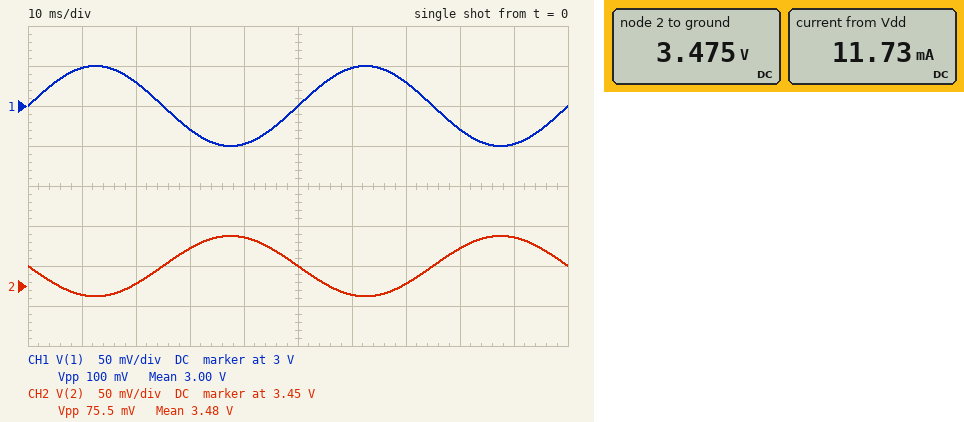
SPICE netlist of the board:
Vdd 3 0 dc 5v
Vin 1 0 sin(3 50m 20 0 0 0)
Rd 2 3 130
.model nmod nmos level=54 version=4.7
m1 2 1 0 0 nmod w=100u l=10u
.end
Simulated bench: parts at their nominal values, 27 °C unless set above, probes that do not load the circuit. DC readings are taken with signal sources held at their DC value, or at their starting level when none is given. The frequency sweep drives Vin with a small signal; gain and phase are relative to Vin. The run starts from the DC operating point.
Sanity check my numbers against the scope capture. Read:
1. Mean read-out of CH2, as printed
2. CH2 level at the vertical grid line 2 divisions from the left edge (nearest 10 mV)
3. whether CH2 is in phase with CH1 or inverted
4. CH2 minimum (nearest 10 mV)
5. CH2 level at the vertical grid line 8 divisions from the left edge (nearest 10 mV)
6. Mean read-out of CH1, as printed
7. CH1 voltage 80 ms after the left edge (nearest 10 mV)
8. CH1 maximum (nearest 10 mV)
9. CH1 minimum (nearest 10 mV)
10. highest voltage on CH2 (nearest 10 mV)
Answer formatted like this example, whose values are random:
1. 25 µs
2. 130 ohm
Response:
1. 3.48 V
2. 3.45 V
3. inverted
4. 3.44 V
5. 3.50 V
6. 3.00 V
7. 2.97 V
8. 3.05 V
9. 2.95 V
10. 3.51 V
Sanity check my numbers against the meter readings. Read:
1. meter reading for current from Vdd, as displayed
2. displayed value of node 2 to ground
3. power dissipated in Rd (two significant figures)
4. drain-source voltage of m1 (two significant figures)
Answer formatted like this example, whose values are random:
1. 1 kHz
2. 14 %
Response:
1. 11.73 mA
2. 3.475 V
3. 18 mW
4. 3.5 V
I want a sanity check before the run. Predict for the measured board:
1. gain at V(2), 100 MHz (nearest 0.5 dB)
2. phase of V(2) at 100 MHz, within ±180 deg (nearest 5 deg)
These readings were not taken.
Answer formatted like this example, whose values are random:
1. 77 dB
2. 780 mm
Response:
1. -2.0 dB
2. 160 deg
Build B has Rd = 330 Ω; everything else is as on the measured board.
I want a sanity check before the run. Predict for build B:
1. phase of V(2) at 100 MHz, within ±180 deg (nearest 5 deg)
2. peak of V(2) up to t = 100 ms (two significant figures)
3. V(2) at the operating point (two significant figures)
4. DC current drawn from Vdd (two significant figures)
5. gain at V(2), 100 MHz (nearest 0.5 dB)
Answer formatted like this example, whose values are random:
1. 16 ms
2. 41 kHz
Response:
1. 125 deg
2. 1.7 V
3. 1.6 V
4. 10 mA
5. -2.5 dB
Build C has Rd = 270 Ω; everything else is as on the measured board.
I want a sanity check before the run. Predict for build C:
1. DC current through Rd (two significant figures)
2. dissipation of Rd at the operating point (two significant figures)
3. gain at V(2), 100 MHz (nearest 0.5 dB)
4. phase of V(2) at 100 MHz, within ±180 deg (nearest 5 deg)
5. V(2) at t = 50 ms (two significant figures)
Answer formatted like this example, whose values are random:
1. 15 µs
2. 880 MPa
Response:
1. 11 mA
2. 33 mW
3. -0.5 dB
4. 140 deg
5. 2.0 V
